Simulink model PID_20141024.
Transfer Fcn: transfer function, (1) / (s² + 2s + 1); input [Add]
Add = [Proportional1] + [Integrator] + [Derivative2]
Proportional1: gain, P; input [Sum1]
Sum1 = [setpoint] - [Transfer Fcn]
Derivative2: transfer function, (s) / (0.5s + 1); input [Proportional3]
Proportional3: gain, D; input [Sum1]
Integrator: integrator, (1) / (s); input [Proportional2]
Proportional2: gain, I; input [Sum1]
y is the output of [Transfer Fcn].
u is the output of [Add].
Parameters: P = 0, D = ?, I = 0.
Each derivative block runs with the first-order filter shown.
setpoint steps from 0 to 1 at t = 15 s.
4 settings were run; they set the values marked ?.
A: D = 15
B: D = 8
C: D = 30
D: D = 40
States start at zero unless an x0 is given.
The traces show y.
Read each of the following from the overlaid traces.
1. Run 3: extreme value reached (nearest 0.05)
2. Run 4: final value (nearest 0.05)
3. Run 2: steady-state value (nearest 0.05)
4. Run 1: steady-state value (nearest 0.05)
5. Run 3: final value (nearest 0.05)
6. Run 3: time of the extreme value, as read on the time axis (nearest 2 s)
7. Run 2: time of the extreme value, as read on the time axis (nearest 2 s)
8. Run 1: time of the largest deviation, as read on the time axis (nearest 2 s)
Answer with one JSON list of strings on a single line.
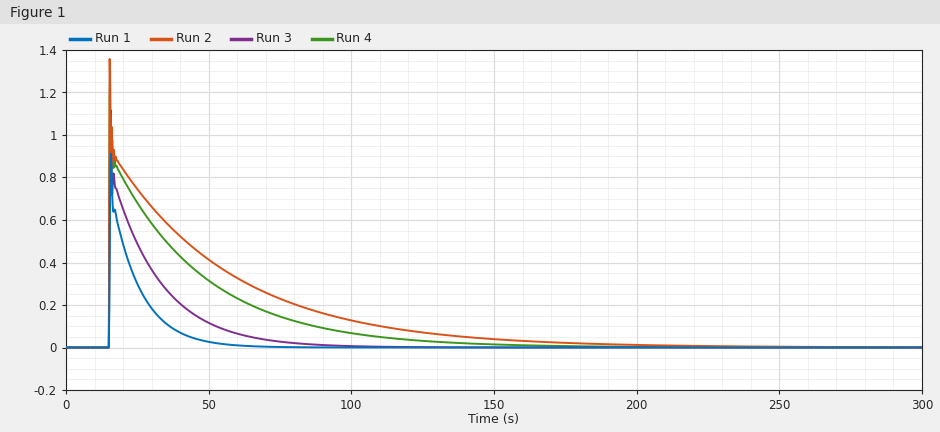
["1.10", "0.00", "0.00", "0.00", "0.00", "16 s", "16 s", "16 s"]
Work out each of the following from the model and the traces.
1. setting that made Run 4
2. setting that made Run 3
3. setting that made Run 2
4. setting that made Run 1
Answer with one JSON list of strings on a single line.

["C", "A", "D", "B"]
